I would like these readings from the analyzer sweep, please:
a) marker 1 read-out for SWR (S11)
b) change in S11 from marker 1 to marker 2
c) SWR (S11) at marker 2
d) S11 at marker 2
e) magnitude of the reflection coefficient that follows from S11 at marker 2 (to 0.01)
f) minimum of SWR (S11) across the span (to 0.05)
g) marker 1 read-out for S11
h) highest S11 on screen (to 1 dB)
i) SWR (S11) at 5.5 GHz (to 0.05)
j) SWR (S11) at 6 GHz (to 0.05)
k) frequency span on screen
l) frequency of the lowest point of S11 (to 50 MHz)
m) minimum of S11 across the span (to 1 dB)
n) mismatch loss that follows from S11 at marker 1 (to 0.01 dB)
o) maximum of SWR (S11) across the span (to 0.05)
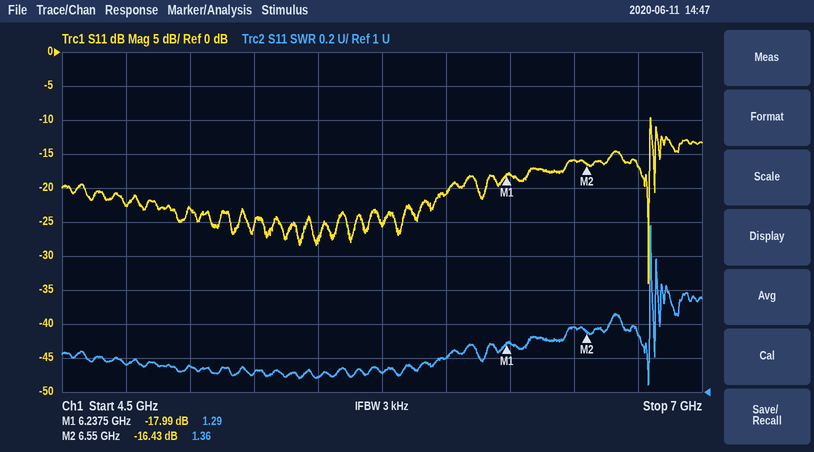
1.29
1.56 dB
1.36
-16.43 dB
0.15
1.05
-17.99 dB
-10 dB
1.10
1.20
2.5 GHz
6.80 GHz
-34 dB
0.07 dB
2.00
